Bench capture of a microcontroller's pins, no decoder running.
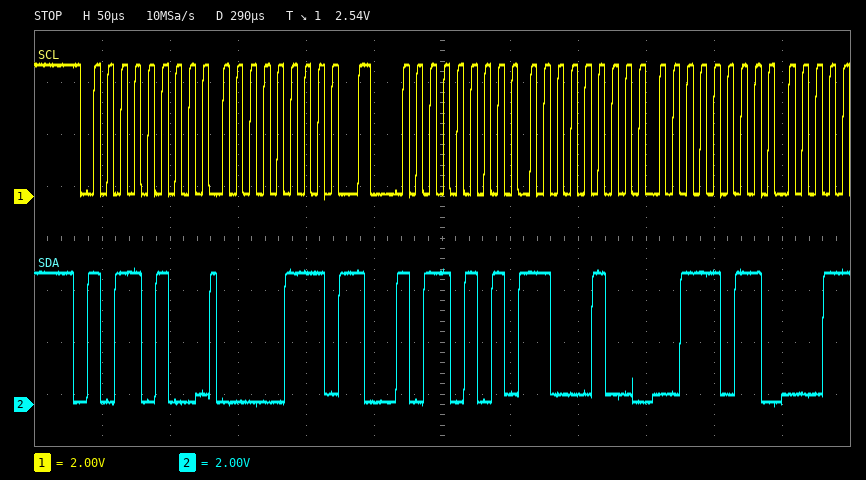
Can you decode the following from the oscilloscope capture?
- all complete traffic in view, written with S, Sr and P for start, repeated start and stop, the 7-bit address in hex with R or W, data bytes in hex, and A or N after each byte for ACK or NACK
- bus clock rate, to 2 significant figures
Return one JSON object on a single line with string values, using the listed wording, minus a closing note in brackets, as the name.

{"all complete traffic in view, written with S, Sr and P for start, repeated start and stop, the 7-bit address in hex with R or W, data bytes in hex, and A or N after each byte for ACK or NACK": "S 5AW A 07 A Sr 5AR A C4 A 3B A", "bus clock rate, to 2 significant figures": "100 kHz"}
